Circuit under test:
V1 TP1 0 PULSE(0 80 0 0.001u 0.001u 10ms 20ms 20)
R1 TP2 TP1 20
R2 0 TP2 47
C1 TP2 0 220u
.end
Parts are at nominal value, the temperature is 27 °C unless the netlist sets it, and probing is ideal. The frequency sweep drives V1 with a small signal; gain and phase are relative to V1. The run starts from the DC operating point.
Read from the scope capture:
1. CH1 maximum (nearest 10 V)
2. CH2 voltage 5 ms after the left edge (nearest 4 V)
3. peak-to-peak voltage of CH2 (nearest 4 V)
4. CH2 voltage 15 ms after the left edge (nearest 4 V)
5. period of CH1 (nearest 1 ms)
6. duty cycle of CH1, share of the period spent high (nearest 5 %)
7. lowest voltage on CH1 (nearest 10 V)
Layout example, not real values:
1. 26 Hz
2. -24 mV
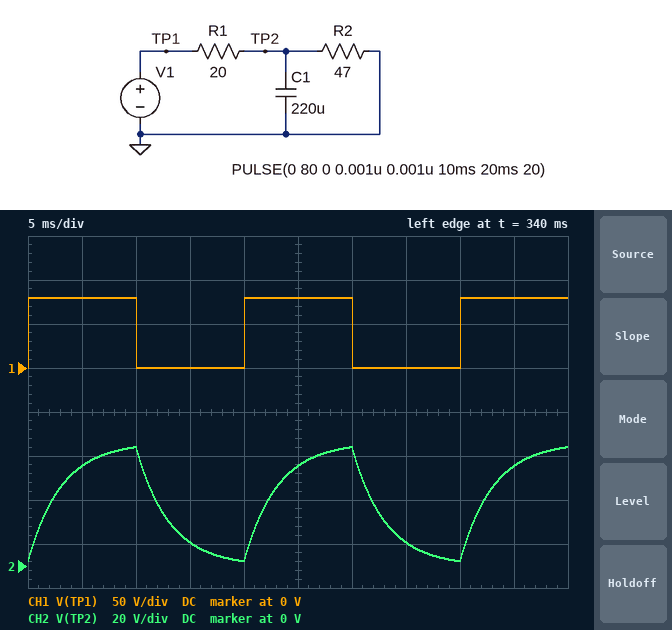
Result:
1. 80 V
2. 44 V
3. 52 V
4. 12 V
5. 20 ms
6. 50 %
7. 0 V
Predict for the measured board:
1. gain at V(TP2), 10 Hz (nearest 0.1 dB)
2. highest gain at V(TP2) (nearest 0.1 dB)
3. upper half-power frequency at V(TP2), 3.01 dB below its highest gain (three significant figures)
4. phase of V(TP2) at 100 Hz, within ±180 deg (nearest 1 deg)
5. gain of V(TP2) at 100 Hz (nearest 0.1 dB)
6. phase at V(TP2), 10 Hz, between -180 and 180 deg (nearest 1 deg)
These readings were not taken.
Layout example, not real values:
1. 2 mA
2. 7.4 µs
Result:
1. -3.2 dB
2. -3.1 dB
3. 51.6 Hz
4. -63 deg
5. -9.9 dB
6. -11 deg
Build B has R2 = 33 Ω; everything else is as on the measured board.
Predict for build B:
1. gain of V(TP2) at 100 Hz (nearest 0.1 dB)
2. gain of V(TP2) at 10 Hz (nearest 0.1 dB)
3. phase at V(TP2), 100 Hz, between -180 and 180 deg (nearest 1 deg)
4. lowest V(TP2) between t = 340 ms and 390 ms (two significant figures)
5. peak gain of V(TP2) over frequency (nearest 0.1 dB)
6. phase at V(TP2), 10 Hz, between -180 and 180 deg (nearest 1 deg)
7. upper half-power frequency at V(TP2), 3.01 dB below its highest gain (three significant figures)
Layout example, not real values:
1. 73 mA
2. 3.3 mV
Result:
1. -10.1 dB
2. -4.2 dB
3. -60 deg
4. 1.3 V
5. -4.1 dB
6. -10 deg
7. 58.1 Hz
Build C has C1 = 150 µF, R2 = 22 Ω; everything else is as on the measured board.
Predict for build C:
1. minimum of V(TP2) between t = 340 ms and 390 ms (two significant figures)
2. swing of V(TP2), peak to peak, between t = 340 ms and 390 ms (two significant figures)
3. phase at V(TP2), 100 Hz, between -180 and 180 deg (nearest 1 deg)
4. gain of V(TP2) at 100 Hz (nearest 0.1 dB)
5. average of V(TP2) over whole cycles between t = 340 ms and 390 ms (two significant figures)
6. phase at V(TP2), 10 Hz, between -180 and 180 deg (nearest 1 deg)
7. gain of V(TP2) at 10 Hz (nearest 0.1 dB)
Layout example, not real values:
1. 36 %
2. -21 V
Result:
1. 72 mV
2. 42 V
3. -45 deg
4. -8.6 dB
5. 21 V
6. -6 deg
7. -5.7 dB
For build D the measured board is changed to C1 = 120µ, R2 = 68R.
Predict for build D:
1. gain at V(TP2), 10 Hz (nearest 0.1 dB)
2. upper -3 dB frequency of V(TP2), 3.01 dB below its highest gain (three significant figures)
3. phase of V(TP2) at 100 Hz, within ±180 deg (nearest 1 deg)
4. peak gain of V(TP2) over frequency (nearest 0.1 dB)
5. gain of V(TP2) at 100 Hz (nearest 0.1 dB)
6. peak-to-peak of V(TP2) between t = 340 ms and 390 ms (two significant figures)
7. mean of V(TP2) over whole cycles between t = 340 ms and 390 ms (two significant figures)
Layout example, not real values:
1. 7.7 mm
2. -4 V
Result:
1. -2.3 dB
2. 85.8 Hz
3. -49 deg
4. -2.2 dB
5. -6.0 dB
6. 61 V
7. 31 V
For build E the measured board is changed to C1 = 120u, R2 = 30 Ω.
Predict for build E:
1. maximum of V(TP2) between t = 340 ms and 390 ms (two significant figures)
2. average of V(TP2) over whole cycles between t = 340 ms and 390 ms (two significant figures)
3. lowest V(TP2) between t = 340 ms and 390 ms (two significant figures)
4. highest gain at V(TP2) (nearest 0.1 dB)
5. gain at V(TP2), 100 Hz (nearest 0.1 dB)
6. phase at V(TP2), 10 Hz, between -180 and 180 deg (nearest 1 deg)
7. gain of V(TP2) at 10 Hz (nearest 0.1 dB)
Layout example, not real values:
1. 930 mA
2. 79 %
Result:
1. 48 V
2. 24 V
3. 46 mV
4. -4.4 dB
5. -7.0 dB
6. -5 deg
7. -4.5 dB
